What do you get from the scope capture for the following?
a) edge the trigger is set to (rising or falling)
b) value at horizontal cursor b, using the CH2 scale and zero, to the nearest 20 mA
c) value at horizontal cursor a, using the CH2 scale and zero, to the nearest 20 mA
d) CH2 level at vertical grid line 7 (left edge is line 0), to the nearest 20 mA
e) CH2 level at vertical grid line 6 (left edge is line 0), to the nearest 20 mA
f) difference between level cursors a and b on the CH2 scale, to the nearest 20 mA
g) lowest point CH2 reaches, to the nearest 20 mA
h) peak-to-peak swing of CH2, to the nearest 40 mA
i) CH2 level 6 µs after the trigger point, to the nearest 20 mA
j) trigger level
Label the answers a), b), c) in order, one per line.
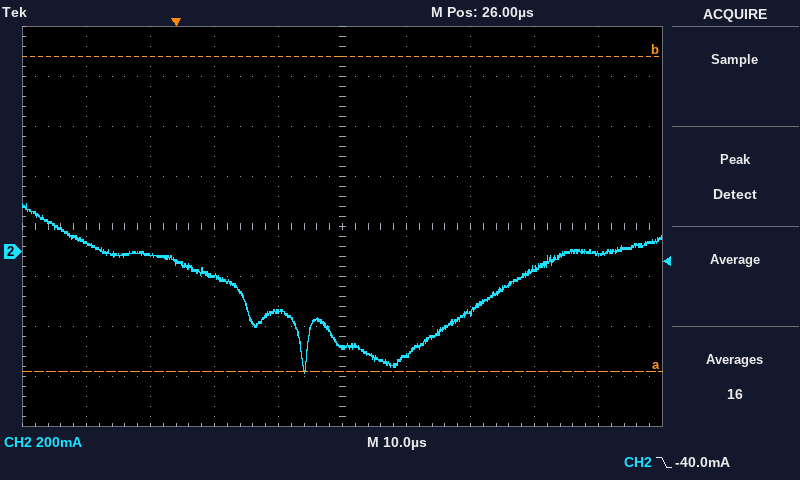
a) falling
b) 780 mA
c) -480 mA
d) -240 mA
e) -420 mA
f) 1.26 A
g) -480 mA
h) 680 mA
i) -100 mA
j) -40.0 mA
